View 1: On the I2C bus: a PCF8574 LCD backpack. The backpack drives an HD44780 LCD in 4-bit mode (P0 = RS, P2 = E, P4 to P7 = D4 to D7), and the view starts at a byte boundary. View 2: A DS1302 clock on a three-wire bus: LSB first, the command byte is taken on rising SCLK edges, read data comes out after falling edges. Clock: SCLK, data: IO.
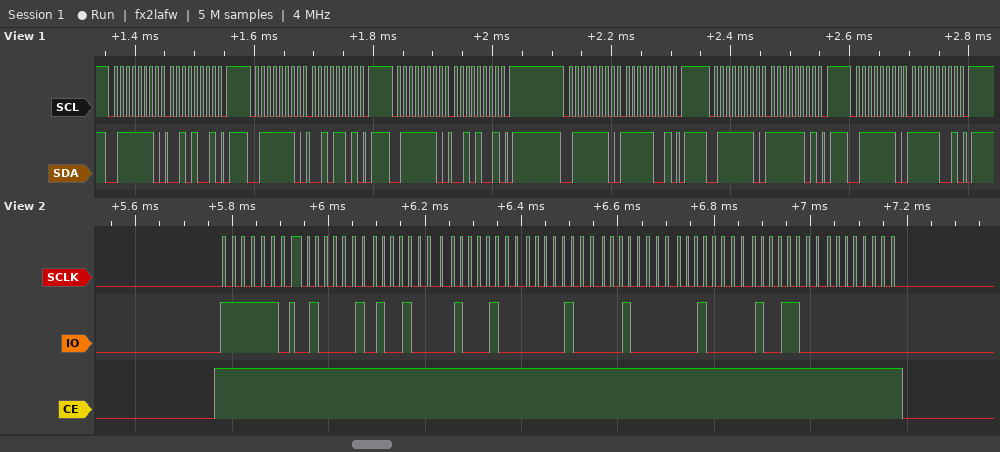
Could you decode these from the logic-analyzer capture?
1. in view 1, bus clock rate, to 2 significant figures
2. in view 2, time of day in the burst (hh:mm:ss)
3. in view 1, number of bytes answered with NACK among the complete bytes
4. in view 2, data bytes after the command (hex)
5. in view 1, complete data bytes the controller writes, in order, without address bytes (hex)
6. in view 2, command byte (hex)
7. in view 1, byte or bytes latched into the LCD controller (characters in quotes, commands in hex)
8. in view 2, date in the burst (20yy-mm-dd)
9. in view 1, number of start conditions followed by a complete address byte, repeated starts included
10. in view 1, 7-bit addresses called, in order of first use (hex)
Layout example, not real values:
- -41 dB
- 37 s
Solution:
- 100 kHz
- 11:09:42
- 0
- 42 09 11 10 04 04 19 00
- 29 2D 29 F9 FD F9
- 0xBF
- '/'
- 2019-04-10
- 6
- 0x3F
